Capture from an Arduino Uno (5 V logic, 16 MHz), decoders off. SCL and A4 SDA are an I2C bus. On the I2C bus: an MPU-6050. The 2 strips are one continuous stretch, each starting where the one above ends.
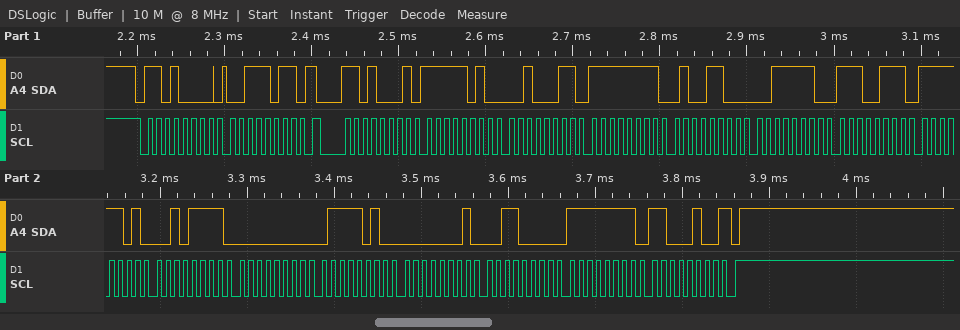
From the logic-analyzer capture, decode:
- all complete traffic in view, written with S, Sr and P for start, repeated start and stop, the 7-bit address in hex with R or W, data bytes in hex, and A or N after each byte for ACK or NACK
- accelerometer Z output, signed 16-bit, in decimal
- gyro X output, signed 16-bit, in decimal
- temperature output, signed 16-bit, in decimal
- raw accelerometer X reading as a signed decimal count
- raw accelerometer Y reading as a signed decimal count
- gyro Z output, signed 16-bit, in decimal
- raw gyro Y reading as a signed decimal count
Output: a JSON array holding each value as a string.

["S 68W A 3B A Sr 68R A FA A 23 A FF A 4C A 3E A E7 A FD A 2F A 00 A 7A A 01 A 30 A FF A C4 N P", "16103", "122", "-721", "-1501", "-180", "-60", "304"]
